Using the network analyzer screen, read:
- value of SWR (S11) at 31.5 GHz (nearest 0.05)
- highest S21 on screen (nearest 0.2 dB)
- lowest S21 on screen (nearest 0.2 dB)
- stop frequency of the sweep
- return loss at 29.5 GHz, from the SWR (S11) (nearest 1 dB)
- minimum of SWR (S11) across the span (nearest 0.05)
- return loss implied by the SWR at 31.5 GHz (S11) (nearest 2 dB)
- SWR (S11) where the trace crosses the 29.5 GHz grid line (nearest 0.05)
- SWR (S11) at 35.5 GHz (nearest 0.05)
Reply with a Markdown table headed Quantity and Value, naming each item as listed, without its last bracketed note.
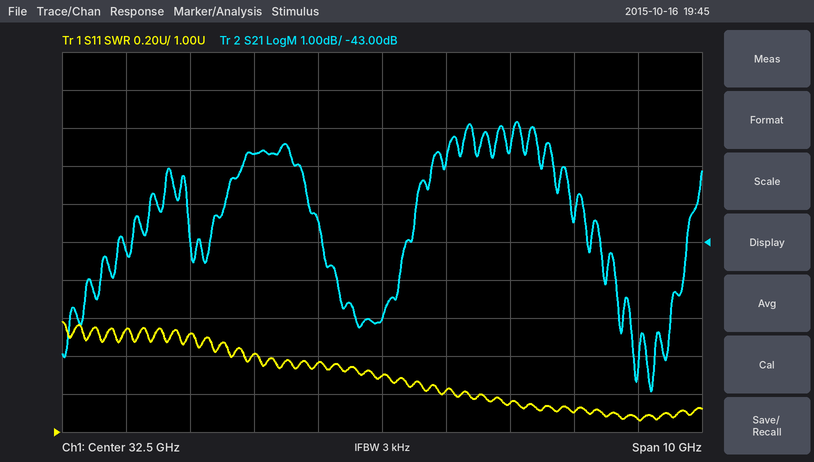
| Quantity | Value |
|---|---|
| value of SWR (S11) at 31.5 GHz | 1.35 |
| highest S21 on screen | -39.8 dB |
| lowest S21 on screen | -47.0 dB |
| stop frequency of the sweep | 37.5 GHz |
| return loss at 29.5 GHz, from the SWR (S11) | 14 dB |
| minimum of SWR (S11) across the span | 1.05 |
| return loss implied by the SWR at 31.5 GHz (S11) | 16 dB |
| SWR (S11) where the trace crosses the 29.5 GHz grid line | 1.50 |
| SWR (S11) at 35.5 GHz | 1.10 |
